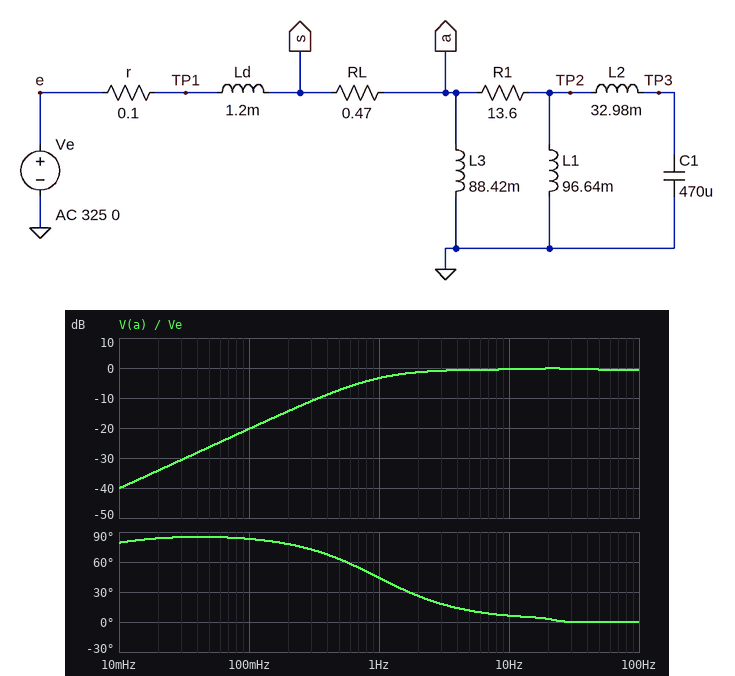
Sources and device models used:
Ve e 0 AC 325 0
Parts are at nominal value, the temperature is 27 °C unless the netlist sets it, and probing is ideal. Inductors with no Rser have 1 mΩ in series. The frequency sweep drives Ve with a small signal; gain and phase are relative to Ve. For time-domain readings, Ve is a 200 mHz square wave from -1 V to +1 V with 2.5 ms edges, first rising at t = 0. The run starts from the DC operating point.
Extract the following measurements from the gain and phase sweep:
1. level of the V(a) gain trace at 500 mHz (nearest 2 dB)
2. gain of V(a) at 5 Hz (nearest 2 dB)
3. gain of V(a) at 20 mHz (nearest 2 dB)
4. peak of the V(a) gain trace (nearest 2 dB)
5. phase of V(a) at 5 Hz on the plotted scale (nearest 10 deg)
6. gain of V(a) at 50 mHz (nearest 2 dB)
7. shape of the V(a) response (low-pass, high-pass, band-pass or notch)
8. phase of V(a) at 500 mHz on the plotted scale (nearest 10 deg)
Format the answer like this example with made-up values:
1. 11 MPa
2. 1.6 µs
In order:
1. -8 dB
2. 0 dB
3. -34 dB
4. 0 dB
5. 10 deg
6. -26 dB
7. high-pass
8. 60 deg
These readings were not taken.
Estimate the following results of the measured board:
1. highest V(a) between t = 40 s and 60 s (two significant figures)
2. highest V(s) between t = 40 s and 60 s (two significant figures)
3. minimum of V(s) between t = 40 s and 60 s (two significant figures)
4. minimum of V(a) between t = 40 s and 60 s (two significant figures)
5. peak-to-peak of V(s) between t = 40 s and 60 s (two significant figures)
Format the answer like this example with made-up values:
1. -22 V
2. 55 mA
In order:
1. 1.9 V
2. 1.1 V
3. -1.1 V
4. -1.9 V
5. 2.3 V
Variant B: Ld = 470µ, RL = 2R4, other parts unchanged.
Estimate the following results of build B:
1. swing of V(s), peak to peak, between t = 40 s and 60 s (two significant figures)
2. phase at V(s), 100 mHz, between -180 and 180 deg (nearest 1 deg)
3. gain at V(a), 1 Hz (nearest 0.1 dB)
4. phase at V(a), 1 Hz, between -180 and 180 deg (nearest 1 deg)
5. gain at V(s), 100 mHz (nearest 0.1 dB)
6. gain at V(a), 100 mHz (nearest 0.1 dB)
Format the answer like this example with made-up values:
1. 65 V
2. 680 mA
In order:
1. 2.0 V
2. 0 deg
3. -13.4 dB
4. 75 deg
5. -0.4 dB
6. -33.1 dB
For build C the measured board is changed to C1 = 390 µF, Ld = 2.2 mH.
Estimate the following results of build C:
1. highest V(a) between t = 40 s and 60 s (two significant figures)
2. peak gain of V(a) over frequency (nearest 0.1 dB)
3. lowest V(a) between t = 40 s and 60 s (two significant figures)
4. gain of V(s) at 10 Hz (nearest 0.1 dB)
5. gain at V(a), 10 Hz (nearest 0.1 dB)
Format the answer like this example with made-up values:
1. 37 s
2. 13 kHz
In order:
1. 1.8 V
2. -0.2 dB
3. -1.8 V
4. -0.3 dB
5. -0.6 dB
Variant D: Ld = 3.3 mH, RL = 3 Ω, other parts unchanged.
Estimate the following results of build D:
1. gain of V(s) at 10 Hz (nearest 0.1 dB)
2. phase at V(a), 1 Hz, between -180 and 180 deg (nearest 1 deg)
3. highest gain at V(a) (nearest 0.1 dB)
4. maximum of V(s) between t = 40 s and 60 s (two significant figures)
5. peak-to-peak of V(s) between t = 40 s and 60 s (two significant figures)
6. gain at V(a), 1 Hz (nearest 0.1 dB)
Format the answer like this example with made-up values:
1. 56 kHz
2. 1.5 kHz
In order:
1. -0.3 dB
2. 77 deg
3. -0.5 dB
4. 980 mV
5. 2.0 V
6. -15.2 dB
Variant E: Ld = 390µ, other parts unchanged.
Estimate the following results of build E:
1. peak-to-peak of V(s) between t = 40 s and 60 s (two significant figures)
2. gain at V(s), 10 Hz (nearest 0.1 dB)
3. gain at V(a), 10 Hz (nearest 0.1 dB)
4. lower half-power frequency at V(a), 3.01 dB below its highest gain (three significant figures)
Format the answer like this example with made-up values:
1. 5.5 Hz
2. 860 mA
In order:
1. 2.3 V
2. -0.1 dB
3. -0.4 dB
4. 1.07 Hz
